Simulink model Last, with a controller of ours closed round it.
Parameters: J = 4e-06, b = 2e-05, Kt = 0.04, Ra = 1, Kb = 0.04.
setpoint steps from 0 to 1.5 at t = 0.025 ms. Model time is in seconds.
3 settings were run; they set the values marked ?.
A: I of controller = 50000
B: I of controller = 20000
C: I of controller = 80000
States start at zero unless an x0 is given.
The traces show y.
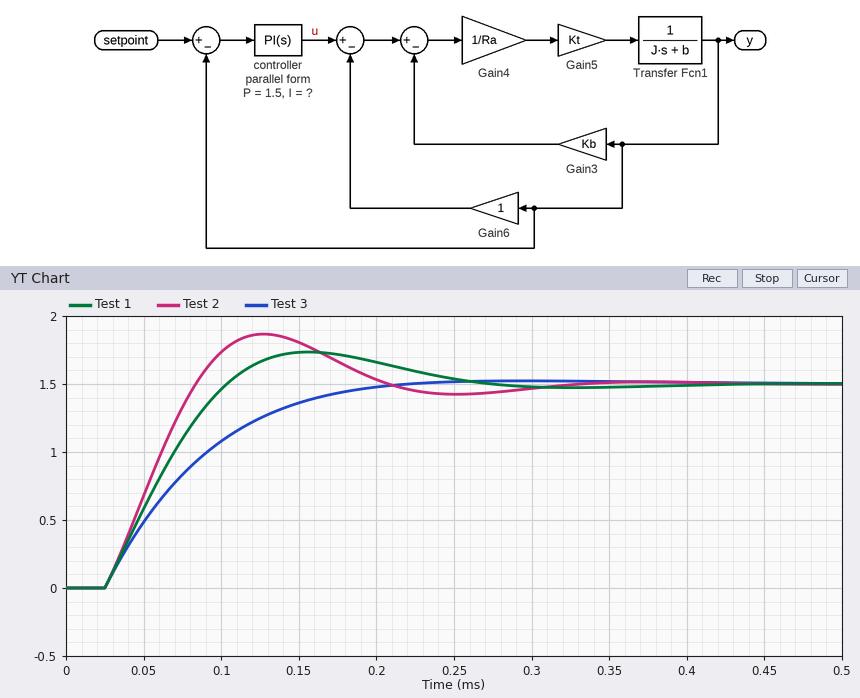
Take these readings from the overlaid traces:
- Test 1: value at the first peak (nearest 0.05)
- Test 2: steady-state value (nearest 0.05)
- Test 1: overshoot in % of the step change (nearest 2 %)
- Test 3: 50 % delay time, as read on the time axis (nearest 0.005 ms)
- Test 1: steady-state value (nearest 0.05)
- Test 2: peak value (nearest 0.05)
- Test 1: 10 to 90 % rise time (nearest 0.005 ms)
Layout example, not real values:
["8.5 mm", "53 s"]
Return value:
["1.75", "1.50", "16 %", "0.070 ms", "1.50", "1.85", "0.060 ms"]
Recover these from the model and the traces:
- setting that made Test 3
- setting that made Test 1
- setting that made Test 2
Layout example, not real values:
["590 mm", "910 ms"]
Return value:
["B", "A", "C"]
